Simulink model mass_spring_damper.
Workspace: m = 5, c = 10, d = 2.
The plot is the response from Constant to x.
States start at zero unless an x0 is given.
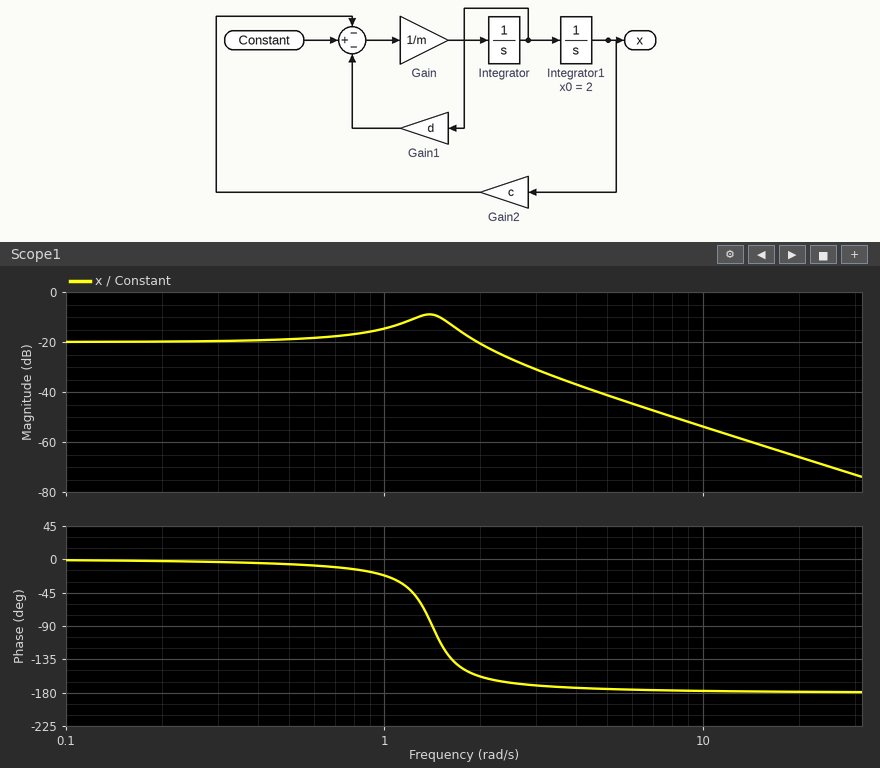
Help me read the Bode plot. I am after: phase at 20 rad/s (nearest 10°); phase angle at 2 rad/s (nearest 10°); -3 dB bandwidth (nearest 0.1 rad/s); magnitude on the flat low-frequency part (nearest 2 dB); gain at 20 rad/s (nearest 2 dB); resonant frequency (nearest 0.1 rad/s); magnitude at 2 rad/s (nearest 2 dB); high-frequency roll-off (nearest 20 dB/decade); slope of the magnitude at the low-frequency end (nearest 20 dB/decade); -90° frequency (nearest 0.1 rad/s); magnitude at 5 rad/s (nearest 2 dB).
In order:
-180°
-160°
2.2 rad/s
-20 dB
-66 dB
1.4 rad/s
-20 dB
-40 dB/decade
0 dB/decade
1.4 rad/s
-42 dB
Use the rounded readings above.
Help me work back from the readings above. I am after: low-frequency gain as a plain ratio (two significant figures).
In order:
0.10
